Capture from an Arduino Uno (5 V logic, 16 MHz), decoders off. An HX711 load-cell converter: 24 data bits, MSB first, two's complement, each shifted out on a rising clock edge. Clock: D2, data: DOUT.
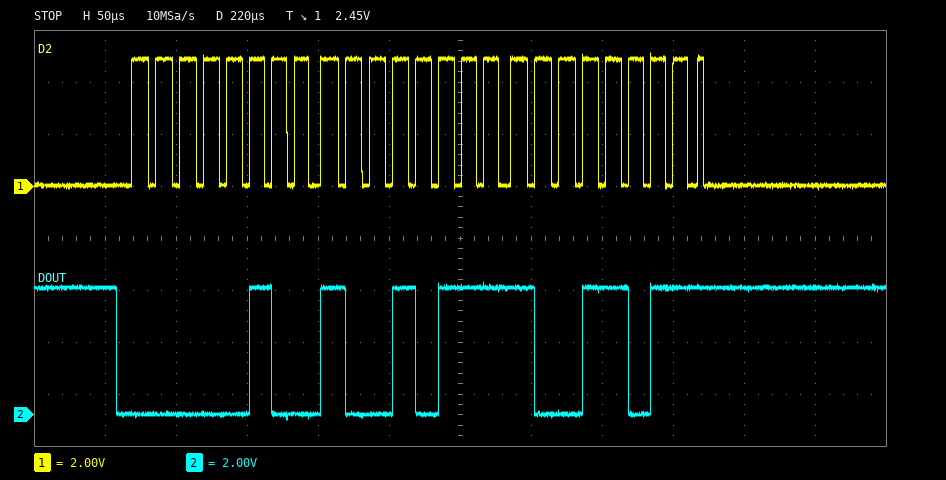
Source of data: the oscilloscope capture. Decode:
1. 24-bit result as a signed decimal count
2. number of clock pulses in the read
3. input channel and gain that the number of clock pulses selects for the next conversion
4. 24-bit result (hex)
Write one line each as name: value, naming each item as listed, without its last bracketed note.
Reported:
24-bit result as a signed decimal count: 300955
number of clock pulses in the read: 25
input channel and gain that the number of clock pulses selects for the next conversion: channel A, gain 128
24-bit result: 0x04979B
